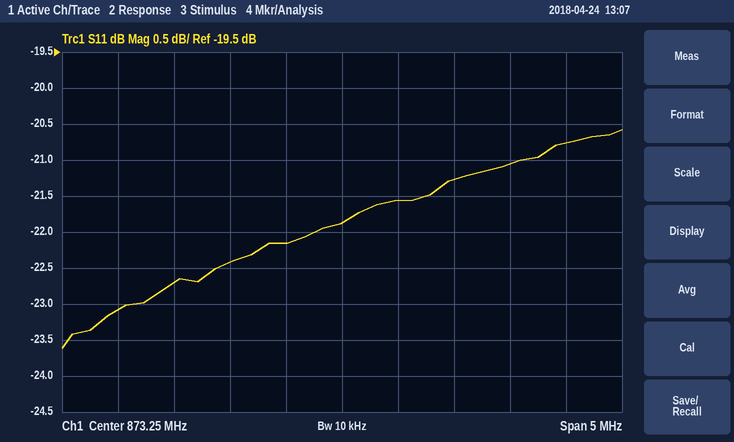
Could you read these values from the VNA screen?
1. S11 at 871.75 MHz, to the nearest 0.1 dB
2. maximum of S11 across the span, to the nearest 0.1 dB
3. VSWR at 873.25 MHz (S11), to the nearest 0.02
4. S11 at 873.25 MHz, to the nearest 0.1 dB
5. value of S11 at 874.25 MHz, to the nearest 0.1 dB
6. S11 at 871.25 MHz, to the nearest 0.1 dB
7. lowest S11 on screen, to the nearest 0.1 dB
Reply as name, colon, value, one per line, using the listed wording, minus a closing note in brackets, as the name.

S11 at 871.75 MHz, to the nearest 0.1 dB: -22.7 dB
maximum of S11 across the span, to the nearest 0.1 dB: -20.6 dB
VSWR at 873.25 MHz (S11), to the nearest 0.02: 1.18
S11 at 873.25 MHz, to the nearest 0.1 dB: -21.9 dB
value of S11 at 874.25 MHz, to the nearest 0.1 dB: -21.3 dB
S11 at 871.25 MHz, to the nearest 0.1 dB: -23.1 dB
lowest S11 on screen, to the nearest 0.1 dB: -23.6 dB
